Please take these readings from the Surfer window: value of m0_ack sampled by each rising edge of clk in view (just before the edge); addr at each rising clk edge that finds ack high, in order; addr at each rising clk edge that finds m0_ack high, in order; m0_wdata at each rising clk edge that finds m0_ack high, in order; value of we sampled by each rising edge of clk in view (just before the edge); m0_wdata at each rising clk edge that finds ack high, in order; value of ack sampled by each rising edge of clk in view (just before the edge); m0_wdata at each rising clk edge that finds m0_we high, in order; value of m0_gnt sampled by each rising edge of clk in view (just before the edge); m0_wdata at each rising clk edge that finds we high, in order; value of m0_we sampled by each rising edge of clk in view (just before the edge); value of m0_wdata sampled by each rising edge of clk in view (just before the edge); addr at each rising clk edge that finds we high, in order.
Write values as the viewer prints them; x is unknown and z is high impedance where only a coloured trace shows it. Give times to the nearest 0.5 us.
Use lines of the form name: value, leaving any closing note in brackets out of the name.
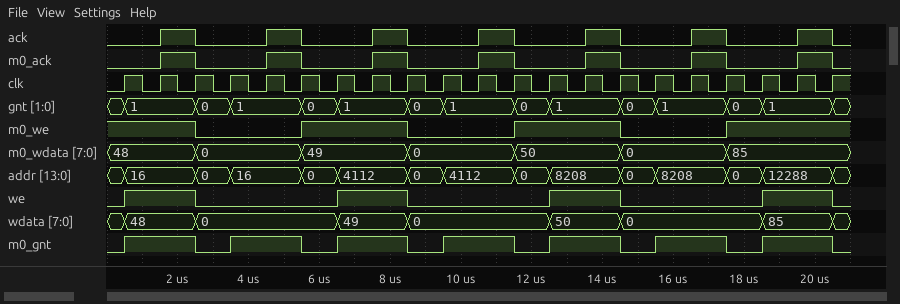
value of m0_ack sampled by each rising edge of clk in view: 0 0 1 0 0 1 0 0 1 0 0 1 0 0 1 0 0 1 0 0 1
addr at each rising clk edge that finds ack high, in order: 16, 16, 4112, 4112, 8208, 8208, 12288
addr at each rising clk edge that finds m0_ack high, in order: 16, 16, 4112, 4112, 8208, 8208, 12288
m0_wdata at each rising clk edge that finds m0_ack high, in order: 48, 0, 49, 0, 50, 0, 85
value of we sampled by each rising edge of clk in view: 0 1 1 0 0 0 0 1 1 0 0 0 0 1 1 0 0 0 0 1 1
m0_wdata at each rising clk edge that finds ack high, in order: 48, 0, 49, 0, 50, 0, 85
value of ack sampled by each rising edge of clk in view: 0 0 1 0 0 1 0 0 1 0 0 1 0 0 1 0 0 1 0 0 1
m0_wdata at each rising clk edge that finds m0_we high, in order: 48, 48, 48, 49, 49, 49, 50, 50, 50, 85, 85, 85
value of m0_gnt sampled by each rising edge of clk in view: 0 1 1 0 1 1 0 1 1 0 1 1 0 1 1 0 1 1 0 1 1
m0_wdata at each rising clk edge that finds we high, in order: 48, 48, 49, 49, 50, 50, 85, 85
value of m0_we sampled by each rising edge of clk in view: 1 1 1 0 0 0 1 1 1 0 0 0 1 1 1 0 0 0 1 1 1
value of m0_wdata sampled by each rising edge of clk in view: 48, 48, 48, 0, 0, 0, 49, 49, 49, 0, 0, 0, 50, 50, 50, 0, 0, 0, 85, 85, 85
addr at each rising clk edge that finds we high, in order: 16, 16, 4112, 4112, 8208, 8208, 12288, 12288
